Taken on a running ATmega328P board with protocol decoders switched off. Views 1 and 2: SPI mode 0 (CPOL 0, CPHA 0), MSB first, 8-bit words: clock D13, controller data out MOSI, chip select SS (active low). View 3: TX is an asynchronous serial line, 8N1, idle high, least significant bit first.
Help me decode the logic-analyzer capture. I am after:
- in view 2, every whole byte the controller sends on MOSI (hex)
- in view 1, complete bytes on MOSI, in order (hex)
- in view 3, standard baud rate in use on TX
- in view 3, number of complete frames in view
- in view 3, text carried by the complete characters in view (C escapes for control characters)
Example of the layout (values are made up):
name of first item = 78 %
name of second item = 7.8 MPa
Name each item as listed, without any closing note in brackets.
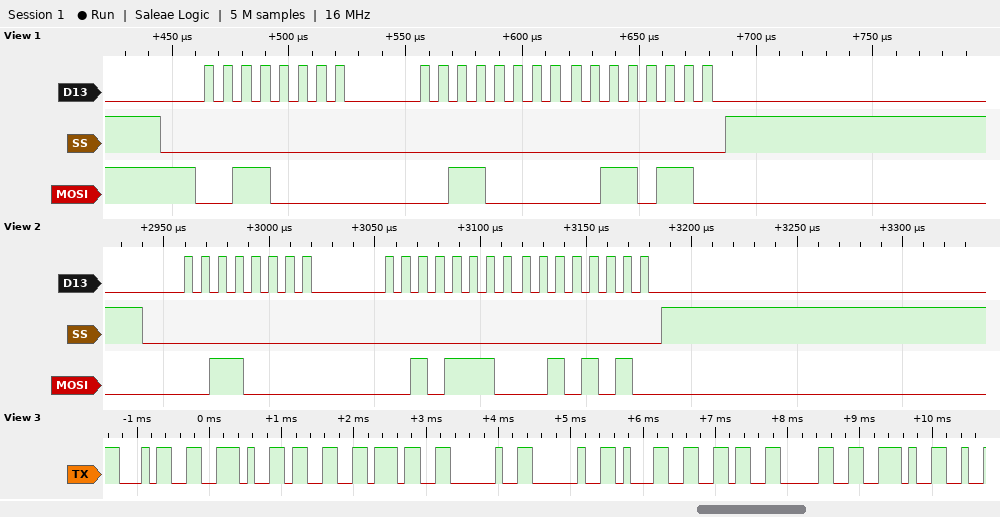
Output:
in view 2, every whole byte the controller sends on MOSI = 30 2E 2A
in view 1, complete bytes on MOSI, in order = 30 30 36
in view 3, standard baud rate in use on TX = 9600 baud
in view 3, number of complete frames in view = 10
in view 3, text carried by the complete characters in view = "4.37  160."
